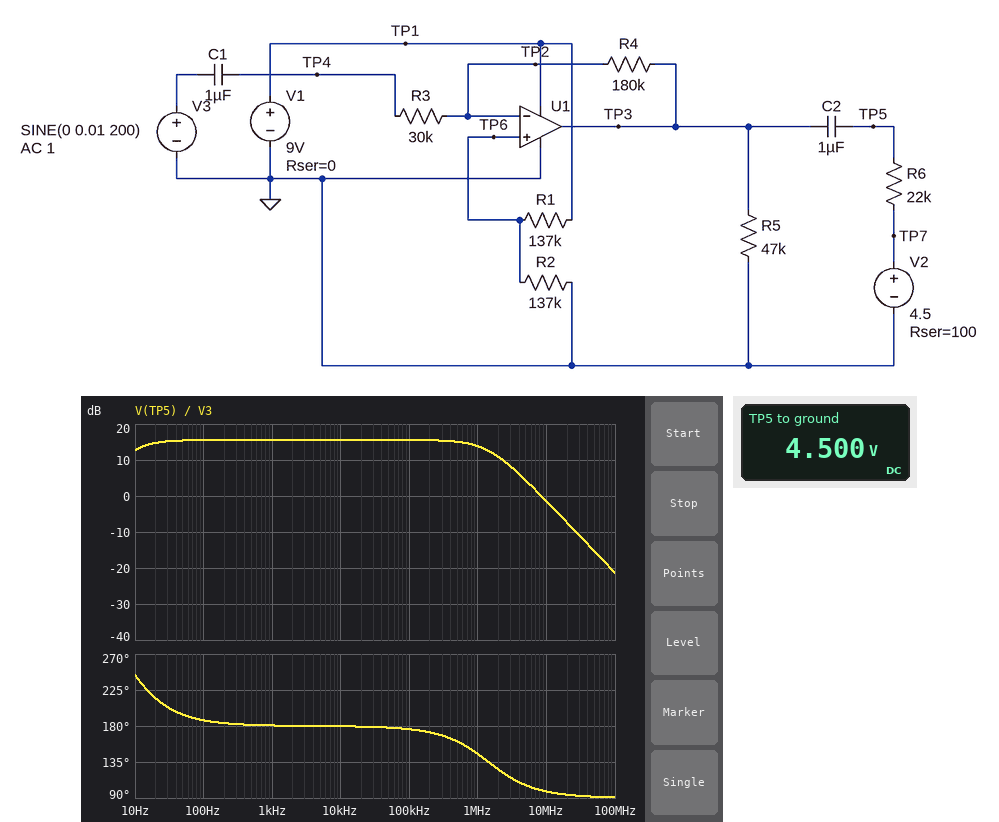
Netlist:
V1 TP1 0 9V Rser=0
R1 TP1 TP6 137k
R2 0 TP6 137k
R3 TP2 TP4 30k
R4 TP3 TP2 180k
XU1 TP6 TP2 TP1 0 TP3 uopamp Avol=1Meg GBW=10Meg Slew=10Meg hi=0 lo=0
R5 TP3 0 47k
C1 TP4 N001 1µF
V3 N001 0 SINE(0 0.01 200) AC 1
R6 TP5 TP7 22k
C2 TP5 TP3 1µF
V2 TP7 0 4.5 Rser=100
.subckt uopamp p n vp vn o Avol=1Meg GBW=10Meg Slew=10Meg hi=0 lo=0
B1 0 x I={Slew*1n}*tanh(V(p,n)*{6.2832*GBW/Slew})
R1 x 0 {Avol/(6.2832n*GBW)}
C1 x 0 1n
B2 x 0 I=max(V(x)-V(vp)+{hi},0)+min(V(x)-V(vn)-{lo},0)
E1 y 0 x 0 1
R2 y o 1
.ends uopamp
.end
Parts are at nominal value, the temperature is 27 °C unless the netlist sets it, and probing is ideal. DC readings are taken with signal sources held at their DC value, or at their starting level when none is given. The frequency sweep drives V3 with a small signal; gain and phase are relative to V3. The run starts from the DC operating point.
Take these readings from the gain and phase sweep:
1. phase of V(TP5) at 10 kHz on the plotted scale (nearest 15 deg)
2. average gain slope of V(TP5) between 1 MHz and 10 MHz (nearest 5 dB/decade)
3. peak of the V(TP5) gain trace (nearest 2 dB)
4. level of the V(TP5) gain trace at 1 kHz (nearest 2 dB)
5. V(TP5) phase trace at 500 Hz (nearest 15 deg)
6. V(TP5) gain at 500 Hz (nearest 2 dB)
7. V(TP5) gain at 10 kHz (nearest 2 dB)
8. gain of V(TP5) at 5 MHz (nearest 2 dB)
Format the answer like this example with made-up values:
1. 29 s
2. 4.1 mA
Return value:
1. 180 deg
2. -15 dB/decade
3. 16 dB
4. 16 dB
5. 180 deg
6. 16 dB
7. 16 dB
8. 4 dB
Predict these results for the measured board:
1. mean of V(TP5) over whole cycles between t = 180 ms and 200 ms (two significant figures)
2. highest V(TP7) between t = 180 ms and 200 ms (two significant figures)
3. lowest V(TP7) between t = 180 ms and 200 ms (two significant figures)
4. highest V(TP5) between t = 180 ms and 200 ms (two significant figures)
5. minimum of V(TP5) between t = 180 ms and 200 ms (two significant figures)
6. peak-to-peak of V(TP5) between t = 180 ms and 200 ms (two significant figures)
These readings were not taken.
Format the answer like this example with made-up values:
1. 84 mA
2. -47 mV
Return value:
1. 4.5 V
2. 4.5 V
3. 4.5 V
4. 4.6 V
5. 4.4 V
6. 120 mV
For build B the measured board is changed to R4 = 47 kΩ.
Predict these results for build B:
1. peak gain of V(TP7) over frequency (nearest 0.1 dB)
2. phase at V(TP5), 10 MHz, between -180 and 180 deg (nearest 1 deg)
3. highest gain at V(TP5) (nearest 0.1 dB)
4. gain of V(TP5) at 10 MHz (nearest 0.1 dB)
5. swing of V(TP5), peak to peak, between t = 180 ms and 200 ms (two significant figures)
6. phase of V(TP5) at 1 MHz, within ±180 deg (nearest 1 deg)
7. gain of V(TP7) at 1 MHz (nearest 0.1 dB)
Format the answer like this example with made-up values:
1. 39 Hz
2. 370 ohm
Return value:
1. -43.0 dB
2. 111 deg
3. 3.9 dB
4. -4.9 dB
5. 31 mV
6. 166 deg
7. -43.3 dB
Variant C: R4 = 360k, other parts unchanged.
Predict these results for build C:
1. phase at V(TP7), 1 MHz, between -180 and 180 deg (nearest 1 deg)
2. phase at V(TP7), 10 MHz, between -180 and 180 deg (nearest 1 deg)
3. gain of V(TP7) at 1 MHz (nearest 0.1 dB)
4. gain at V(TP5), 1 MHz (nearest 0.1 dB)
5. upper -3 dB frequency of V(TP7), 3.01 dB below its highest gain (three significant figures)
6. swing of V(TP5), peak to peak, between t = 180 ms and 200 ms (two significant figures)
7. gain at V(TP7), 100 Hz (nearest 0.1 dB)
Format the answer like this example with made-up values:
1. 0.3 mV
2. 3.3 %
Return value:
1. 128 deg
2. 94 deg
3. -29.6 dB
4. 17.3 dB
5. 769 kHz
6. 240 mV
7. -25.3 dB
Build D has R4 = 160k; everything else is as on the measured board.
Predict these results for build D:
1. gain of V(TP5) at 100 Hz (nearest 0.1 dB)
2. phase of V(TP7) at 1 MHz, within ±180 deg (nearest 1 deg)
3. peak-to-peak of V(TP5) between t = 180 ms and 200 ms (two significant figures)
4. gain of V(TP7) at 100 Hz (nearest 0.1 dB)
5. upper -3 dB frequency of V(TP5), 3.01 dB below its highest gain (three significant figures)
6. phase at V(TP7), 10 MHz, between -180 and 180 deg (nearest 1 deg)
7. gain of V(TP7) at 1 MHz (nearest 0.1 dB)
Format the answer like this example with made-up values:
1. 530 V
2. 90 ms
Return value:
1. 14.5 dB
2. 148 deg
3. 110 mV
4. -32.4 dB
5. 1.58 MHz
6. 99 deg
7. -33.8 dB
